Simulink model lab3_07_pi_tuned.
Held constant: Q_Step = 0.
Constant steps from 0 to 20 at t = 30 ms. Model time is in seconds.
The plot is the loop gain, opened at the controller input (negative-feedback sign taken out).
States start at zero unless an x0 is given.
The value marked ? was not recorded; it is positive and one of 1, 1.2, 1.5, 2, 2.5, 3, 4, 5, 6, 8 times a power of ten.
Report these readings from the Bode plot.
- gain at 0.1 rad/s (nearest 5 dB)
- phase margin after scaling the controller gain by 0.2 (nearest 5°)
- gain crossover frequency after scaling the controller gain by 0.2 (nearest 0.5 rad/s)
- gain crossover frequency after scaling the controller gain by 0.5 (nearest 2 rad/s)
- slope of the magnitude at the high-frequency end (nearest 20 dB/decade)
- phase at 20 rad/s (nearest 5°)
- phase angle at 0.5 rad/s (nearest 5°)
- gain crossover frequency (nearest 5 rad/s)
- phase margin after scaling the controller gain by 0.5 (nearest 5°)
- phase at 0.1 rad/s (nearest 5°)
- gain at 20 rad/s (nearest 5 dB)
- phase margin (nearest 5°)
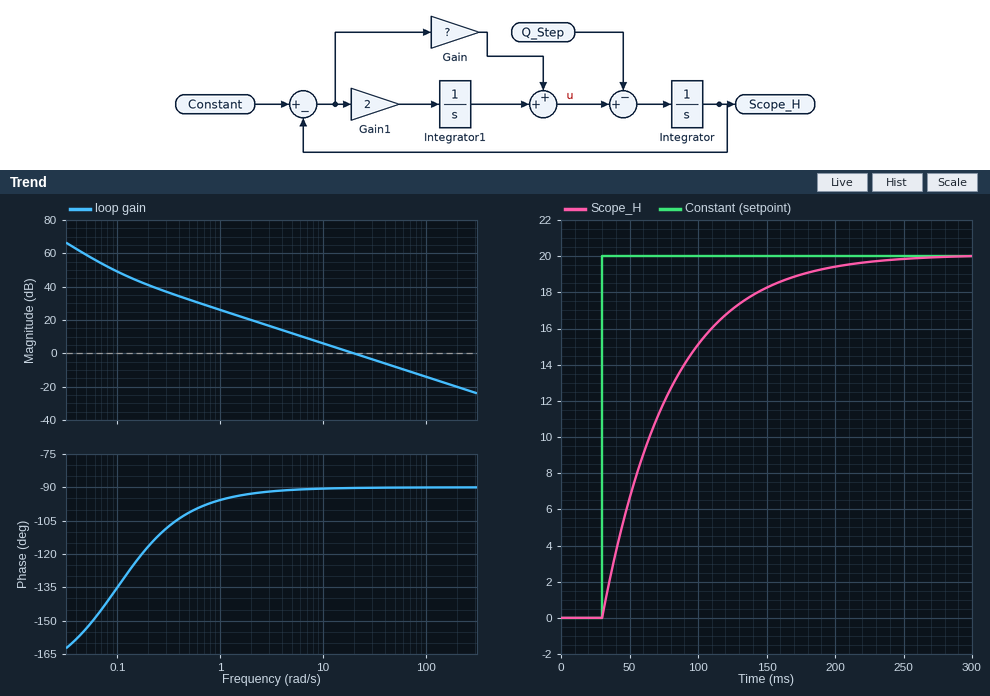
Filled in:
50 dB
90°
4.0 rad/s
10 rad/s
-20 dB/decade
-90°
-100°
20 rad/s
90°
-135°
0 dB
90°
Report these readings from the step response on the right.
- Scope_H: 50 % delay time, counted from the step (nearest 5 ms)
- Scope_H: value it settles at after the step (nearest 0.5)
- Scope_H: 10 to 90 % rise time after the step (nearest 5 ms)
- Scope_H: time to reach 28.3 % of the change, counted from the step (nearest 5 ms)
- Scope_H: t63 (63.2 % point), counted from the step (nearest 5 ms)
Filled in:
35 ms
20.0
110 ms
15 ms
50 ms
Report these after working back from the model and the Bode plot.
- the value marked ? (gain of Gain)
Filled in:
20
